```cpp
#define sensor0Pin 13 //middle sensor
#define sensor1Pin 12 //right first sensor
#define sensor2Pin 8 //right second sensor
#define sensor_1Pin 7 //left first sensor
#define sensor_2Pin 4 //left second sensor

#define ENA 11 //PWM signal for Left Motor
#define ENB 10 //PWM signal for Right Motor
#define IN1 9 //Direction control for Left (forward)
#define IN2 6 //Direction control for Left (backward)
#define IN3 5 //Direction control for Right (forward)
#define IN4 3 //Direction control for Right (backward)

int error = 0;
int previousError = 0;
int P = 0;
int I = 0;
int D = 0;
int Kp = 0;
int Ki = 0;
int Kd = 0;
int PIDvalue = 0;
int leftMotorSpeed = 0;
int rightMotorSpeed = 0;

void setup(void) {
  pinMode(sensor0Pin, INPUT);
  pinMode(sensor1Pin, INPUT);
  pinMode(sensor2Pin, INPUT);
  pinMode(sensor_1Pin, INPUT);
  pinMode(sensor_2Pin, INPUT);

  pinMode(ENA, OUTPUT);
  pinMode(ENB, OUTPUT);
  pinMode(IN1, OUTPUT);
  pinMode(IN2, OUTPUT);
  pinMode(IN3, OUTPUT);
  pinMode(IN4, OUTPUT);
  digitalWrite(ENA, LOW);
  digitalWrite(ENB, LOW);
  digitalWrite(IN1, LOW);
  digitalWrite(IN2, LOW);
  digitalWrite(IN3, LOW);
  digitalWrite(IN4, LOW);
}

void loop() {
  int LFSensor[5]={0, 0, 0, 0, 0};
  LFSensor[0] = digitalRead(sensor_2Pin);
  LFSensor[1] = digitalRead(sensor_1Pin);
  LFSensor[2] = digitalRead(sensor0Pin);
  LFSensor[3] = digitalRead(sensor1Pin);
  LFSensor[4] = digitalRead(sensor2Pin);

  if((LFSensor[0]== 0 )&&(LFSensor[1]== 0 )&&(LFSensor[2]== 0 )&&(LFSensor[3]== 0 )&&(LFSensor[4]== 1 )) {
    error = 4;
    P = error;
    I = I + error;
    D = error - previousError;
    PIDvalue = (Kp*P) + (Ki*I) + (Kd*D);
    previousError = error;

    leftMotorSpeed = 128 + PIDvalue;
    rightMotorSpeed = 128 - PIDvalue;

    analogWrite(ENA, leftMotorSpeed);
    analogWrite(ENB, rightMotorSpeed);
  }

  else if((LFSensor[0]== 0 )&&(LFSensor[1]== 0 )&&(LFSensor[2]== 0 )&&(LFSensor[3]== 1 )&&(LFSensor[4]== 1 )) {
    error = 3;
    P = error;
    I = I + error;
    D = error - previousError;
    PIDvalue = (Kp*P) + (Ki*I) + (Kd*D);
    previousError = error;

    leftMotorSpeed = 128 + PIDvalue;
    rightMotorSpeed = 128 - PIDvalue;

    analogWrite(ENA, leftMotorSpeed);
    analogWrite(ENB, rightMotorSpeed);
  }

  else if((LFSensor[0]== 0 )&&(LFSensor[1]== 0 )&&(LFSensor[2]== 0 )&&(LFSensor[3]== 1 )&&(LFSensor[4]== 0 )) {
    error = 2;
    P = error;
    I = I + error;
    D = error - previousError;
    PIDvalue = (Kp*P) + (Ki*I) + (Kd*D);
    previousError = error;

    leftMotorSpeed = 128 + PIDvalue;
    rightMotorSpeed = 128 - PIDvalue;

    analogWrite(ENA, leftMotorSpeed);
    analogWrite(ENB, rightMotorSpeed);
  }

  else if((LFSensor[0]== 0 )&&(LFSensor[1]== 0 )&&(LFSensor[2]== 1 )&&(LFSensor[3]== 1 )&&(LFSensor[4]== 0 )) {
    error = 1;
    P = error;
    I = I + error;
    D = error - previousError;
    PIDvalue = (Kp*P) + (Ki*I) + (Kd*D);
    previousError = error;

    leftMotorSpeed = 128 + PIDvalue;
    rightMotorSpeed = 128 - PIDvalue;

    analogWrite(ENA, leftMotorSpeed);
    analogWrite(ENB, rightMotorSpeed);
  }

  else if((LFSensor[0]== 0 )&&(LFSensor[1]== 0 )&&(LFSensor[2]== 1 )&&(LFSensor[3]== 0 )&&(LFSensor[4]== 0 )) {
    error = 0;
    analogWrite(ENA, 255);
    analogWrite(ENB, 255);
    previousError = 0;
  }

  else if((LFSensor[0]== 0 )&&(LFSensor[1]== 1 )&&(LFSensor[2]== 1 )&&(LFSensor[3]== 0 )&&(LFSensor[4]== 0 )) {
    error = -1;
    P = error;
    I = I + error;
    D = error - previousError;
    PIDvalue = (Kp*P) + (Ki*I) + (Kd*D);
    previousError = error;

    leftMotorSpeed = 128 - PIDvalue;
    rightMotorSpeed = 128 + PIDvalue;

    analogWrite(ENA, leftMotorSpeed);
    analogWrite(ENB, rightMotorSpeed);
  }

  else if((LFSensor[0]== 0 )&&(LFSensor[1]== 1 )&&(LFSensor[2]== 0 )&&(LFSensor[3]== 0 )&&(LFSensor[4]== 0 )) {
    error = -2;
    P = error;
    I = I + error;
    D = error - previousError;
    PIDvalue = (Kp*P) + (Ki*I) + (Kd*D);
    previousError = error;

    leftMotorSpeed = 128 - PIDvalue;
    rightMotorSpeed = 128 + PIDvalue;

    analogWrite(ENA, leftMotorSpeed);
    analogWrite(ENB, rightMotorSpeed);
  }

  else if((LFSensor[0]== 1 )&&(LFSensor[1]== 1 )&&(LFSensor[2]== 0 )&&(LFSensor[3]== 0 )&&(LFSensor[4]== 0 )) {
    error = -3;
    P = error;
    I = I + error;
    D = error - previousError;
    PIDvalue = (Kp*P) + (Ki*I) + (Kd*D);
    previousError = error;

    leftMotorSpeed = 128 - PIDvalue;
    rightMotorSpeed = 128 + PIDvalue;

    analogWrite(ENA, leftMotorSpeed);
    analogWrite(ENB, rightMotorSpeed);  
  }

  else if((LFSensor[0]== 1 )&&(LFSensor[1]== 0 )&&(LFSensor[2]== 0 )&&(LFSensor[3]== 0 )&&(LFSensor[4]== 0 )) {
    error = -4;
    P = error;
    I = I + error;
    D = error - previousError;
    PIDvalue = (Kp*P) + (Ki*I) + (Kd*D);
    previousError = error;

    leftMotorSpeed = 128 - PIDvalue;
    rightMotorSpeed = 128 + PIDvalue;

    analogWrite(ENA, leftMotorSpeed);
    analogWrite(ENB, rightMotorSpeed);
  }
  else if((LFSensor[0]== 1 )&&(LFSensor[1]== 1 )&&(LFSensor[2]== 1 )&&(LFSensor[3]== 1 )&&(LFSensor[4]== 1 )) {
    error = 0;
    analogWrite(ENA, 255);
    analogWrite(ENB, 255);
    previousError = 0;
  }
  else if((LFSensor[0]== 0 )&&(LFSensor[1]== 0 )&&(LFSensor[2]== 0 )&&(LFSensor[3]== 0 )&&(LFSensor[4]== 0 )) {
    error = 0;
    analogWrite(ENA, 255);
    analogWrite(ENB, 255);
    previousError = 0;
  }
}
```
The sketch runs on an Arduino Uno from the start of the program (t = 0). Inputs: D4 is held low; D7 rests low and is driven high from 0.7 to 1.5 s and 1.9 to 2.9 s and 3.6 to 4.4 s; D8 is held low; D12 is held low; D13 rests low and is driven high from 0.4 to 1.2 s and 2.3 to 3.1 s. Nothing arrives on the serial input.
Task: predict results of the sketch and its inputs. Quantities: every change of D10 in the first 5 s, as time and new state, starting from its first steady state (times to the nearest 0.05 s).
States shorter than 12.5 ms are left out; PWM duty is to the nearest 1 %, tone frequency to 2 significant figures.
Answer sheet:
0 s high; 0.7 s PWM 50 %; 1.5 s high; 1.9 s PWM 50 %; 2.9 s high; 3.6 s PWM 50 %; 4.4 s high
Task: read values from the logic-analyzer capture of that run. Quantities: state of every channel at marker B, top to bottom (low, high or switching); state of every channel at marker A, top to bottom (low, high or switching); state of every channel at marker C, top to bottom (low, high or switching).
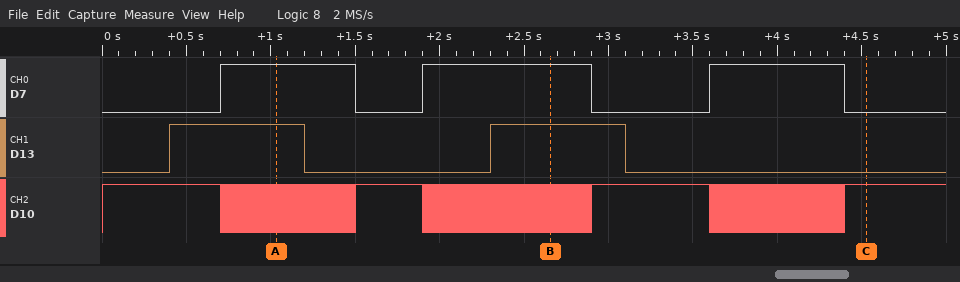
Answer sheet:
D7 high, D13 high, D10 switching
D7 high, D13 high, D10 switching
D7 low, D13 low, D10 high
